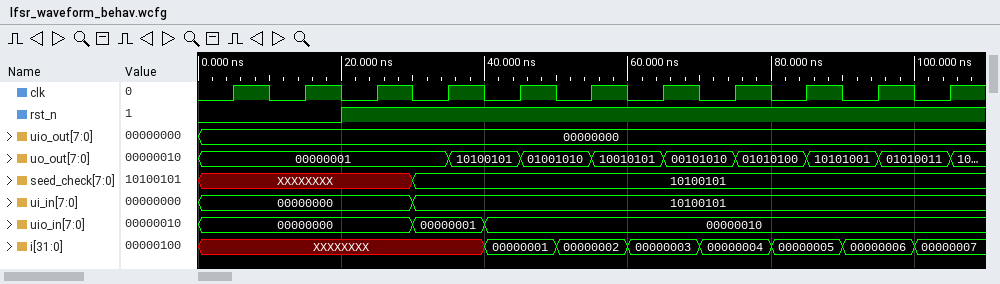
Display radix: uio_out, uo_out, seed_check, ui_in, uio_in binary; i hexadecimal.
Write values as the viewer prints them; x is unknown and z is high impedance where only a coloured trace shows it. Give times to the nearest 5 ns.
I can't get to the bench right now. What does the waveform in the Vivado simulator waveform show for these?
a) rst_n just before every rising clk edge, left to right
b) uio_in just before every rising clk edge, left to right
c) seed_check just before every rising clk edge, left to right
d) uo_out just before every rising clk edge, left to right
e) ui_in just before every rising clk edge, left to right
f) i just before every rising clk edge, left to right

0 0 1 1 1 1 1 1 1 1 1
00000000, 00000000, 00000000, 00000001, 00000010, 00000010, 00000010, 00000010, 00000010, 00000010, 00000010
XXXXXXXX, XXXXXXXX, XXXXXXXX, 10100101, 10100101, 10100101, 10100101, 10100101, 10100101, 10100101, 10100101
00000001, 00000001, 00000001, 00000001, 10100101, 01001010, 10010101, 00101010, 01010100, 10101001, 01010011
00000000, 00000000, 00000000, 10100101, 10100101, 10100101, 10100101, 10100101, 10100101, 10100101, 10100101
XXXXXXXX, XXXXXXXX, XXXXXXXX, XXXXXXXX, 00000001, 00000002, 00000003, 00000004, 00000005, 00000006, 00000007
